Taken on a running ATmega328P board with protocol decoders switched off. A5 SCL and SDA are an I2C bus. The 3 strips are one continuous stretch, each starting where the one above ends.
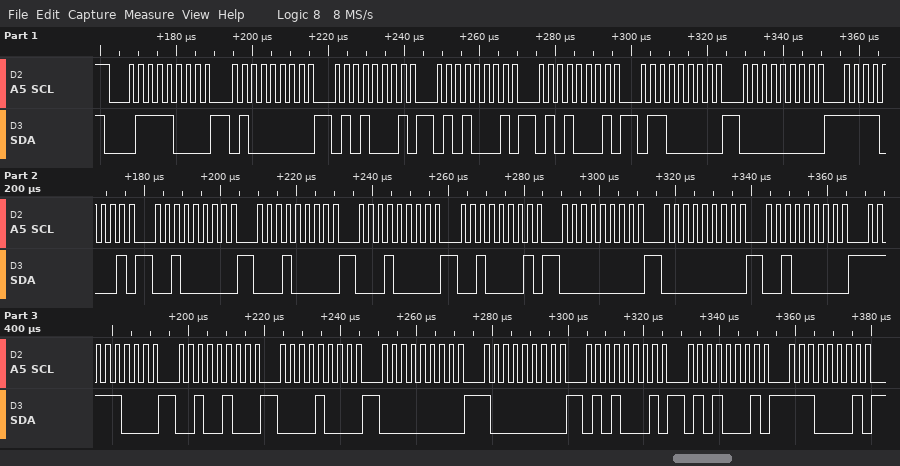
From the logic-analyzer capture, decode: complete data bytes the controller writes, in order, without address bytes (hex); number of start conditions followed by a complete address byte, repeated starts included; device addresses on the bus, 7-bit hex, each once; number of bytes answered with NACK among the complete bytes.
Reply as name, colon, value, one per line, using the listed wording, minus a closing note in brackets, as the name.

complete data bytes the controller writes, in order, without address bytes: 40 51 51 51 60 00 F1 20 10 10 21 00 00 20 F8 24 08 00 80 51 51 E1
number of start conditions followed by a complete address byte, repeated starts included: 1
device addresses on the bus, 7-bit hex, each once: 0x3C
number of bytes answered with NACK among the complete bytes: 0
